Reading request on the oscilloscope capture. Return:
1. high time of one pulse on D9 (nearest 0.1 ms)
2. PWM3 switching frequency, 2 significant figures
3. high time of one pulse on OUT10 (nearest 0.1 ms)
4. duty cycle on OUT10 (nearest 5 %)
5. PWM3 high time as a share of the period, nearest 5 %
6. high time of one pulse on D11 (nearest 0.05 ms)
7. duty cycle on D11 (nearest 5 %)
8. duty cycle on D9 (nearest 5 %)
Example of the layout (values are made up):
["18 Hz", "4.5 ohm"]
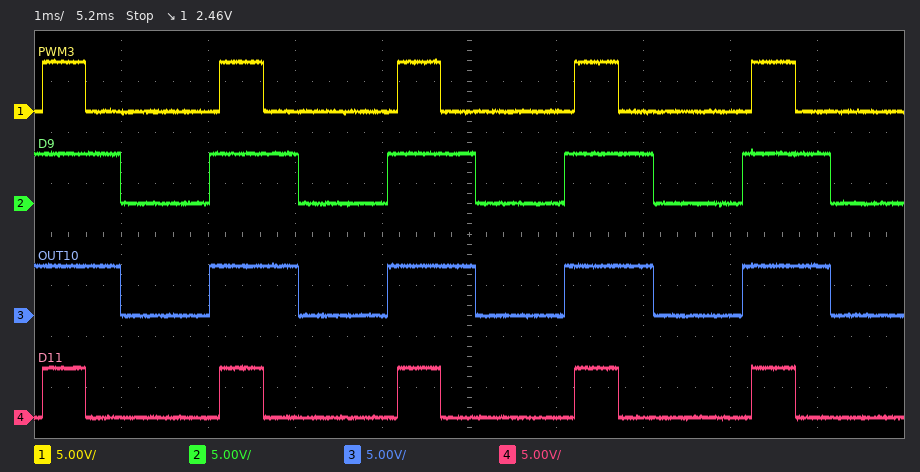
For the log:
["1.0 ms", "490 Hz", "1.0 ms", "50 %", "25 %", "0.50 ms", "25 %", "50 %"]
